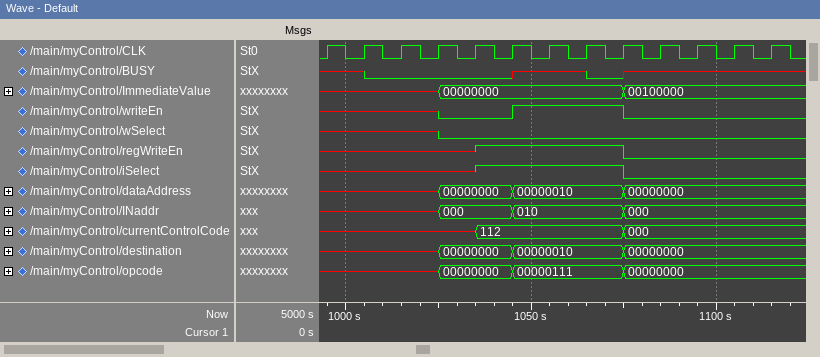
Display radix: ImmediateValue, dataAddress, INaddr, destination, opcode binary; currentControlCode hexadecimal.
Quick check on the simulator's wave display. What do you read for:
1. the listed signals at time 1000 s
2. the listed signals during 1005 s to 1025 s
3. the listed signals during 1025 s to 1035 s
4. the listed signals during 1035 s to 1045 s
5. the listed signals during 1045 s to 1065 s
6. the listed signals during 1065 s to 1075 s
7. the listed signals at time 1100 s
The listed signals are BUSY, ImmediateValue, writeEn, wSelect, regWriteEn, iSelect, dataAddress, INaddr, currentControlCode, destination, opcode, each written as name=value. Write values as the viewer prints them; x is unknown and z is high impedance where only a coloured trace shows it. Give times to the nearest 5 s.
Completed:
BUSY=x, ImmediateValue=x, writeEn=x, wSelect=x, regWriteEn=x, iSelect=x, dataAddress=x, INaddr=x, currentControlCode=x, destination=x, opcode=x
BUSY=0, ImmediateValue=x, writeEn=x, wSelect=x, regWriteEn=x, iSelect=x, dataAddress=x, INaddr=x, currentControlCode=x, destination=x, opcode=x
BUSY=0, ImmediateValue=00000000, writeEn=0, wSelect=0, regWriteEn=x, iSelect=x, dataAddress=00000000, INaddr=000, currentControlCode=x, destination=00000000, opcode=00000000
BUSY=0, ImmediateValue=00000000, writeEn=0, wSelect=0, regWriteEn=1, iSelect=1, dataAddress=00000000, INaddr=000, currentControlCode=112, destination=00000000, opcode=00000000
BUSY=x, ImmediateValue=00000000, writeEn=1, wSelect=0, regWriteEn=1, iSelect=1, dataAddress=00000010, INaddr=010, currentControlCode=112, destination=00000010, opcode=00000111
BUSY=0, ImmediateValue=00000000, writeEn=1, wSelect=0, regWriteEn=1, iSelect=1, dataAddress=00000010, INaddr=010, currentControlCode=112, destination=00000010, opcode=00000111
BUSY=x, ImmediateValue=00100000, writeEn=0, wSelect=0, regWriteEn=0, iSelect=0, dataAddress=00000000, INaddr=000, currentControlCode=000, destination=00000000, opcode=00000000
